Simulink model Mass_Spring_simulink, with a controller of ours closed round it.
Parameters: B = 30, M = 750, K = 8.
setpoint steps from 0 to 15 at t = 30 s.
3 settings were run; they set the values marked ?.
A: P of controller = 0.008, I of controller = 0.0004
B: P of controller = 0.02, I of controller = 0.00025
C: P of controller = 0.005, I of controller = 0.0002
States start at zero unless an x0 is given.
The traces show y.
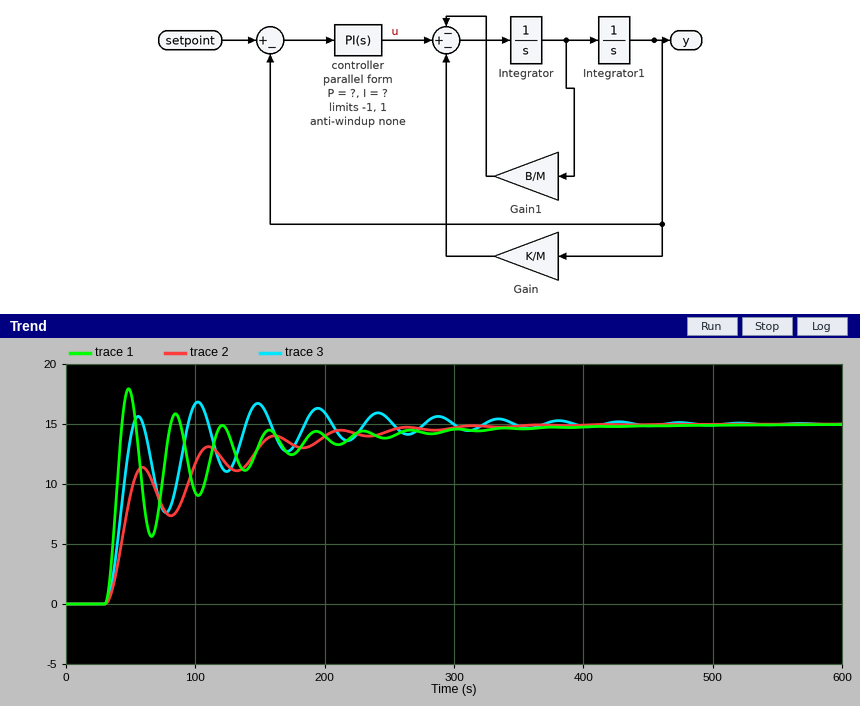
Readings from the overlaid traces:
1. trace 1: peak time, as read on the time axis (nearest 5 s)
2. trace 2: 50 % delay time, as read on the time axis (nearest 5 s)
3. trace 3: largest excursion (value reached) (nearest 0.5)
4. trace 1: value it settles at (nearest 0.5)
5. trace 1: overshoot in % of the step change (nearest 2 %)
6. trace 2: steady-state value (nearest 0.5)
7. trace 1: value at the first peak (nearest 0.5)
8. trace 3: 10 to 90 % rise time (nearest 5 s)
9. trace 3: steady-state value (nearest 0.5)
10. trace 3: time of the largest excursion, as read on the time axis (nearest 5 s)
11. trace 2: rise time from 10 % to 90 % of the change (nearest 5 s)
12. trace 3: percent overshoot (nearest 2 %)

50 s
45 s
17.0
15.0
20 %
15.0
18.0
15 s
15.0
100 s
115 s
12 %
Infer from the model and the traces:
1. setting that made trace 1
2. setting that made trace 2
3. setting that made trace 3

B
C
A
